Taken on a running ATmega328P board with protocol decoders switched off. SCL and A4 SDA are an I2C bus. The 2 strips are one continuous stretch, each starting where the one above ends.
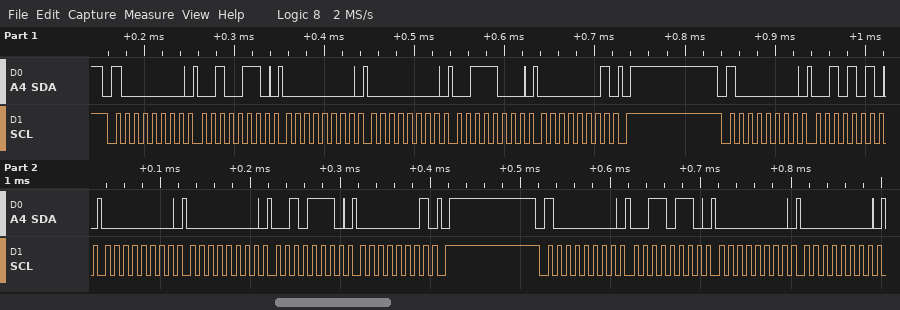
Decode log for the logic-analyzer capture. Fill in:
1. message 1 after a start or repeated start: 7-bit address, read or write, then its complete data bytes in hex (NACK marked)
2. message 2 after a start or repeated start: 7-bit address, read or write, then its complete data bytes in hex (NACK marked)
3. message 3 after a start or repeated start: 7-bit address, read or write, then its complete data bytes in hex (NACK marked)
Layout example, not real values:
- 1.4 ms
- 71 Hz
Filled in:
- 0x40 write: 26 00 00 38 01
- 0x40 write: 2A 00 00 2E 01
- 0x40 write: 36 00 00
